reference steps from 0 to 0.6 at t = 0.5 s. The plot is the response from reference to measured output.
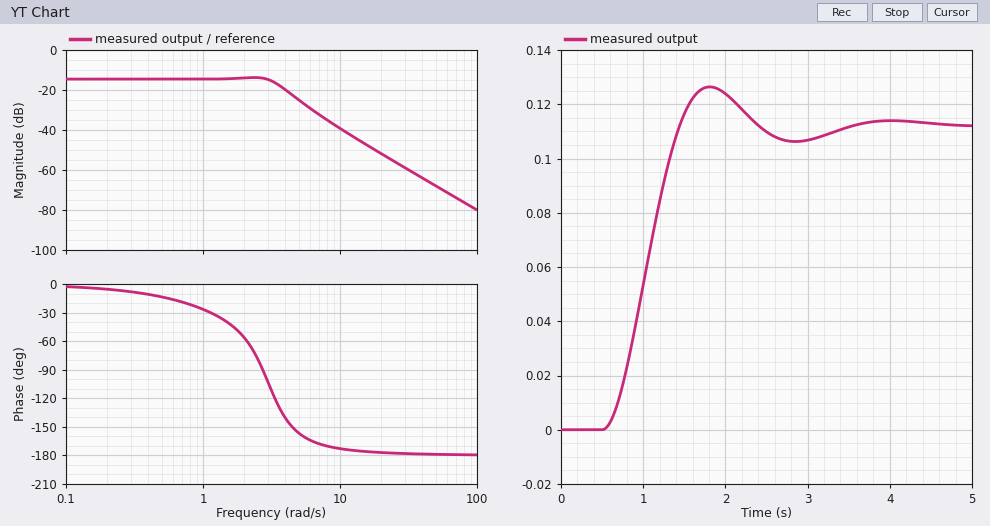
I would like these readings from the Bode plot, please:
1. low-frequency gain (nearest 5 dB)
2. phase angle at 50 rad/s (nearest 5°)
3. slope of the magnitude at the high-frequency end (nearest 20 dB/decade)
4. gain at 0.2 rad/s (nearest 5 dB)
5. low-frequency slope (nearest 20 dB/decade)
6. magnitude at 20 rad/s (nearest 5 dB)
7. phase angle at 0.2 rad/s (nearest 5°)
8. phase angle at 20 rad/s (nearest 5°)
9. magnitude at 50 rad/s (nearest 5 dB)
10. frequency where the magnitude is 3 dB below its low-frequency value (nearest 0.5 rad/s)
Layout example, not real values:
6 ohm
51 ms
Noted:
-15 dB
-180°
-40 dB/decade
-15 dB
0 dB/decade
-50 dB
-5°
-175°
-70 dB
3.5 rad/s
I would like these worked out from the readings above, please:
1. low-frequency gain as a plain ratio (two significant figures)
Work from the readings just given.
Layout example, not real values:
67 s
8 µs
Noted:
0.18
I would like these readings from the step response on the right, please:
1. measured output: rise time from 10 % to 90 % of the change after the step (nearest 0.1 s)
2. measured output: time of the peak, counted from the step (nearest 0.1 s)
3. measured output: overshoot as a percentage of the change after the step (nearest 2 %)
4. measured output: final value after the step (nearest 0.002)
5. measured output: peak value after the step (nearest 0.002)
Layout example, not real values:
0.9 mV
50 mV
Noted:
0.6 s
1.3 s
12 %
0.112
0.126
